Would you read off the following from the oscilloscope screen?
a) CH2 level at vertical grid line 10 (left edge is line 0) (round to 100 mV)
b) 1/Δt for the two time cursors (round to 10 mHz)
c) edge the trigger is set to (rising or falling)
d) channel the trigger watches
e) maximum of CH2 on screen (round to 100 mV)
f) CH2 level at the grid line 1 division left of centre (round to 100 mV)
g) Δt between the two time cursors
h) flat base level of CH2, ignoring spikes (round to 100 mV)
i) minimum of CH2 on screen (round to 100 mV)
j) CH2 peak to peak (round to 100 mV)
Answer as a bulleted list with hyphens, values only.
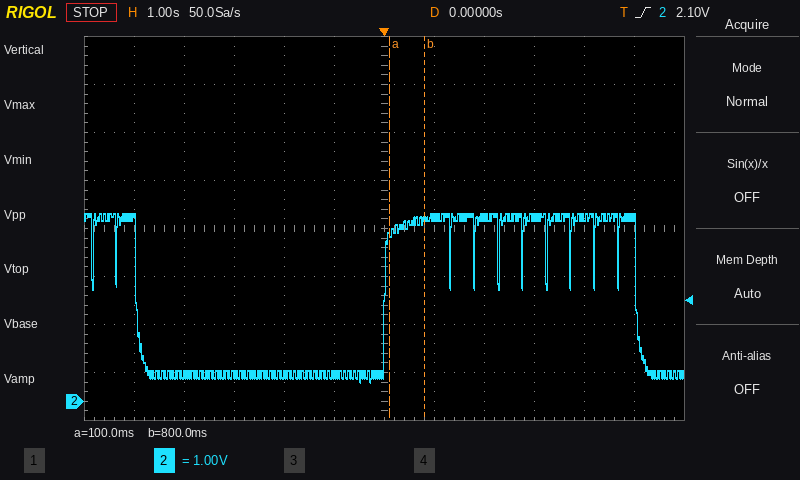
- 3.8 V
- 1.43 Hz
- rising
- CH2
- 3.9 V
- 600 mV
- 700 ms
- 600 mV
- 400 mV
- 3.5 V
